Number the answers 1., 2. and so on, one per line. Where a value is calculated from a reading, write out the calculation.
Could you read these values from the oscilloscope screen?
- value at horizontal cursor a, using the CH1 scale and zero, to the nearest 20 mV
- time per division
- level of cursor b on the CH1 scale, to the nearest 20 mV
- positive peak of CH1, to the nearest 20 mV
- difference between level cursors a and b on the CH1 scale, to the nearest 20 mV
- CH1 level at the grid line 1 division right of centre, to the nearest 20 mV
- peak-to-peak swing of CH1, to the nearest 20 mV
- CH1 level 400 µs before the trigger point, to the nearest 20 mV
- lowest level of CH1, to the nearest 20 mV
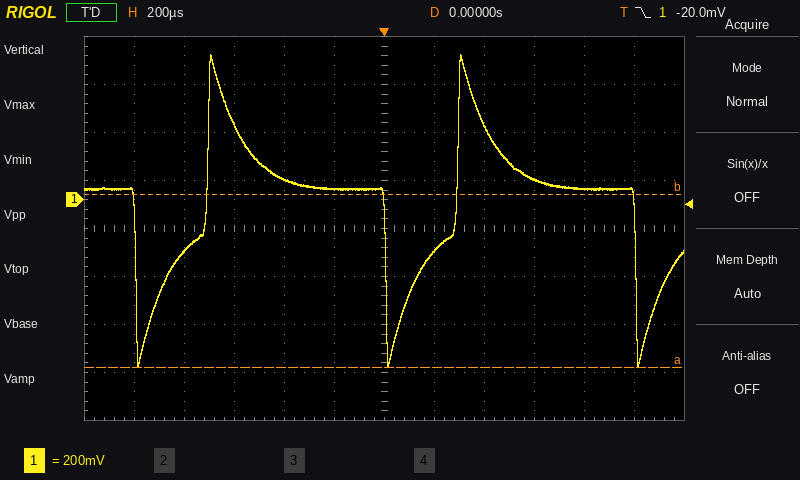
1. -700 mV
2. 200 µs
3. 20 mV
4. 600 mV
5. 720 mV
6. -220 mV
7. 600 mV − (-700 mV) = 1.30 V
8. 80 mV
9. -700 mV
